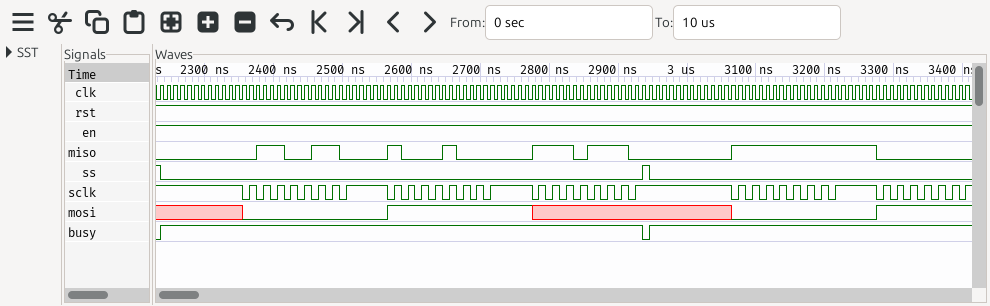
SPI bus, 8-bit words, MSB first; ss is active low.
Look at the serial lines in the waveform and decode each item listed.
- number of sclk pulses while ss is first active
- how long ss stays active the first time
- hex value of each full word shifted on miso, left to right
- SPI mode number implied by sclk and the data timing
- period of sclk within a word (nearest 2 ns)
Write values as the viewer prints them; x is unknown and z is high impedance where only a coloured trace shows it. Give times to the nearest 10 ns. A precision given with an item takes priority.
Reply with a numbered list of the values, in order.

1. 24
2. 700 ns
3. 66, 88, EE, FF
4. 3
5. 20 ns
